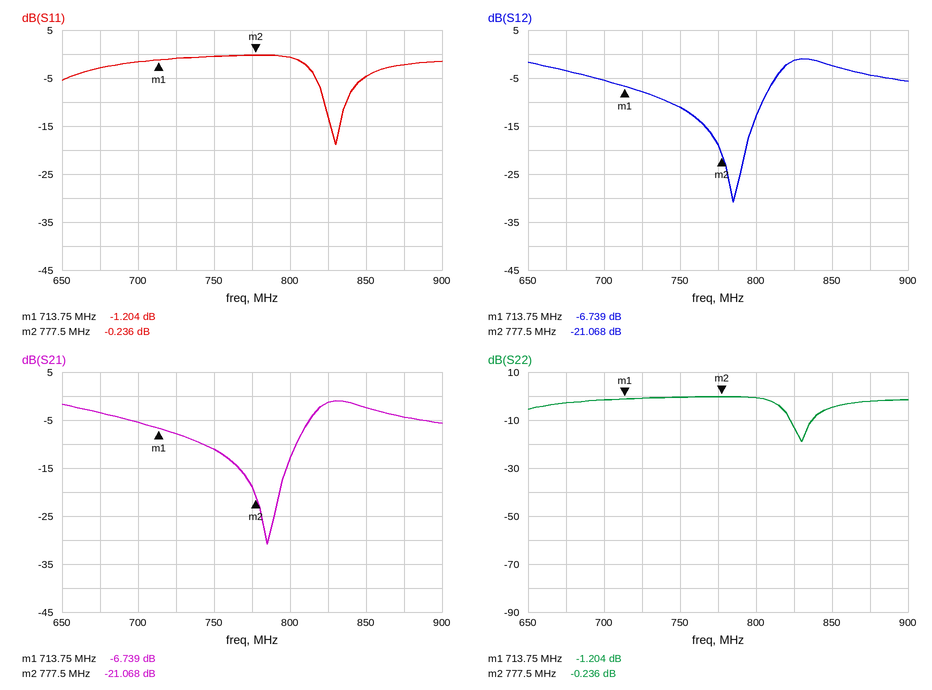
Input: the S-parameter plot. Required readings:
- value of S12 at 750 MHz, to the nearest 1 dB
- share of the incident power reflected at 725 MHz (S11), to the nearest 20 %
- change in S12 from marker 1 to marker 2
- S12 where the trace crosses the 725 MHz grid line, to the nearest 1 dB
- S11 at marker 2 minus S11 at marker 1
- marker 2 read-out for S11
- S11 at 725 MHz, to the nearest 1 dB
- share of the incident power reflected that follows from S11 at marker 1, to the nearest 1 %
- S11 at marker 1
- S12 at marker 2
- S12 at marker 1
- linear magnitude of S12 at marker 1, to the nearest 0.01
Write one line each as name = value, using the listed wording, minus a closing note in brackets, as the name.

value of S12 at 750 MHz, to the nearest 1 dB = -11 dB
share of the incident power reflected at 725 MHz (S11), to the nearest 20 % = 80 %
change in S12 from marker 1 to marker 2 = -14.329 dB
S12 where the trace crosses the 725 MHz grid line, to the nearest 1 dB = -8 dB
S11 at marker 2 minus S11 at marker 1 = 0.968 dB
marker 2 read-out for S11 = -0.236 dB
S11 at 725 MHz, to the nearest 1 dB = -1 dB
share of the incident power reflected that follows from S11 at marker 1, to the nearest 1 % = 76 %
S11 at marker 1 = -1.204 dB
S12 at marker 2 = -21.068 dB
S12 at marker 1 = -6.739 dB
linear magnitude of S12 at marker 1, to the nearest 0.01 = 0.46
